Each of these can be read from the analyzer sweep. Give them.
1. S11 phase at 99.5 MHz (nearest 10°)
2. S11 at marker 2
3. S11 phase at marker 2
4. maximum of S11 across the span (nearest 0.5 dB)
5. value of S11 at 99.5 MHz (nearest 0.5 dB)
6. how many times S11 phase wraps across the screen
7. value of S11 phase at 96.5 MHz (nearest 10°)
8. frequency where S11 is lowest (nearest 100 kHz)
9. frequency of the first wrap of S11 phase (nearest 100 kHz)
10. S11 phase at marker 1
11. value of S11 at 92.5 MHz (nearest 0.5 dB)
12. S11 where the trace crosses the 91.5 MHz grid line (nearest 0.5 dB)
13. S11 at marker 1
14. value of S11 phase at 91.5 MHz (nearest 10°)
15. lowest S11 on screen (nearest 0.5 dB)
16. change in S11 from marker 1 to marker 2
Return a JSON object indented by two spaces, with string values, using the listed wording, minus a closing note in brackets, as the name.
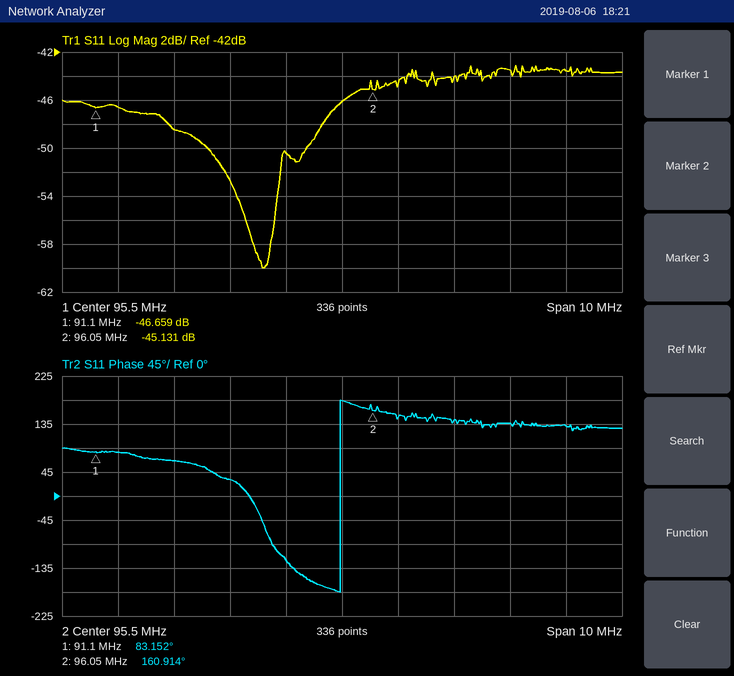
{
  "S11 phase at 99.5 MHz": "130°",
  "S11 at marker 2": "-45.131 dB",
  "S11 phase at marker 2": "160.914°",
  "maximum of S11 across the span": "-43.0 dB",
  "value of S11 at 99.5 MHz": "-43.5 dB",
  "how many times S11 phase wraps across the screen": "1",
  "value of S11 phase at 96.5 MHz": "150°",
  "frequency where S11 is lowest": "94.1 MHz",
  "frequency of the first wrap of S11 phase": "95.5 MHz",
  "S11 phase at marker 1": "83.152°",
  "value of S11 at 92.5 MHz": "-48.5 dB",
  "S11 where the trace crosses the 91.5 MHz grid line": "-46.5 dB",
  "S11 at marker 1": "-46.659 dB",
  "value of S11 phase at 91.5 MHz": "80°",
  "lowest S11 on screen": "-60.0 dB",
  "change in S11 from marker 1 to marker 2": "1.528 dB"
}
